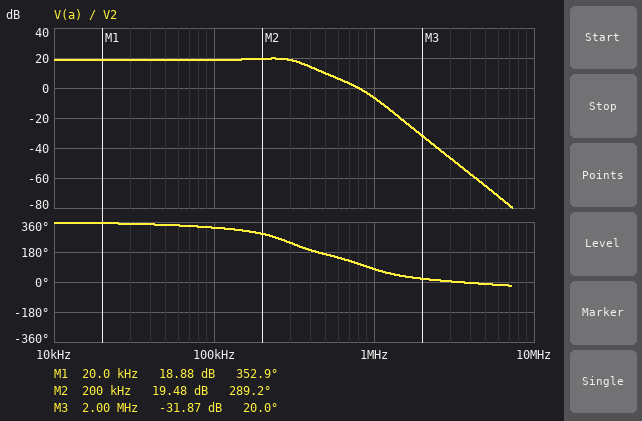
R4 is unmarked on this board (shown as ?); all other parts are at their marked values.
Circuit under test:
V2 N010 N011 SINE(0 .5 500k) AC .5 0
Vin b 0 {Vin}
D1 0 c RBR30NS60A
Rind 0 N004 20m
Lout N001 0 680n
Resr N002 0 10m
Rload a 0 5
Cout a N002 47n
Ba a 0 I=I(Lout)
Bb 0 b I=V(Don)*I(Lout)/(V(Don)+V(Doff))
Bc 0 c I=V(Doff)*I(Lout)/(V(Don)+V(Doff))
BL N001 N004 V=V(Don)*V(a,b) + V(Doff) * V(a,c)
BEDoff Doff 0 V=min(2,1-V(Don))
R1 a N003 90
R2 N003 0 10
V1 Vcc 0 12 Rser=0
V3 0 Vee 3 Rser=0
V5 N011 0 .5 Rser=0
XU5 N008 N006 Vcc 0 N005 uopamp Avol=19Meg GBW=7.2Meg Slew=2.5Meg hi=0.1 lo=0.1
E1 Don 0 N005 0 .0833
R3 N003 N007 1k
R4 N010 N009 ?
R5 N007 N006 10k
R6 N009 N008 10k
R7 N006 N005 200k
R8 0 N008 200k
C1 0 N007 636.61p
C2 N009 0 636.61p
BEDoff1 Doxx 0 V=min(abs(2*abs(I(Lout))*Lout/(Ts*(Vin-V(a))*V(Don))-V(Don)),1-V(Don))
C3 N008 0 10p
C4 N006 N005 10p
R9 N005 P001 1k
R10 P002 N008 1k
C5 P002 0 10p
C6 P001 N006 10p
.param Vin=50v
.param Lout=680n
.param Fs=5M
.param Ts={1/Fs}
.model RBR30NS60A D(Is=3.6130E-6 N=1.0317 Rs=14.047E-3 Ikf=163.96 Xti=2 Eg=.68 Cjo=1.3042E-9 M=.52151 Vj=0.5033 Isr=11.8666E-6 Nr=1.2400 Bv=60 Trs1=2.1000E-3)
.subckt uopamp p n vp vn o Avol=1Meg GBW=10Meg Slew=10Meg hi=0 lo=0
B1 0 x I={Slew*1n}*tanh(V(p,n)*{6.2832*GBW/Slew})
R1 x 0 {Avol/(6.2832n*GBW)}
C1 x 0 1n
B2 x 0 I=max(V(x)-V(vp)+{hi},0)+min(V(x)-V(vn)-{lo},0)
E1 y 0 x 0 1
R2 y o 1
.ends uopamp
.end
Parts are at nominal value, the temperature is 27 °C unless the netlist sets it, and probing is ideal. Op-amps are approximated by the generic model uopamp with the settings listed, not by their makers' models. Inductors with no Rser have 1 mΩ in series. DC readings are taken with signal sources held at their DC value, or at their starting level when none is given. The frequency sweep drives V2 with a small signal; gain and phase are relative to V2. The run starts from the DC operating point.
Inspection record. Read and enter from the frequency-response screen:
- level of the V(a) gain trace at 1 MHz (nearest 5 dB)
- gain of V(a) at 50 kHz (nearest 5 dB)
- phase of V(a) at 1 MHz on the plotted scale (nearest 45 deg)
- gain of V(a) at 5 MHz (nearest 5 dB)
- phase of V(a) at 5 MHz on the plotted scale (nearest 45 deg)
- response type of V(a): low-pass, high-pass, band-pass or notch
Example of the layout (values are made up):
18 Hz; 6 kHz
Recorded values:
-5 dB; 20 dB; 90 deg; -65 dB; 0 deg; low-pass
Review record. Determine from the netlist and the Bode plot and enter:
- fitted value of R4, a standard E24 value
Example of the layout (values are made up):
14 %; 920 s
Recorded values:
1.6 kΩ
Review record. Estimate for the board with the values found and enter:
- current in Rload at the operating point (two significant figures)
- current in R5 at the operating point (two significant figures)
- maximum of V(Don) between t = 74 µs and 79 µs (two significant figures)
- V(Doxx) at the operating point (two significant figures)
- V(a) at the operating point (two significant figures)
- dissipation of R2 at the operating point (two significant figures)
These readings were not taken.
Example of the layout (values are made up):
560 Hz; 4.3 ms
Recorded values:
870 mA; 3.3 µA; 120 mV; 94 mV; 4.4 V; 19 mW
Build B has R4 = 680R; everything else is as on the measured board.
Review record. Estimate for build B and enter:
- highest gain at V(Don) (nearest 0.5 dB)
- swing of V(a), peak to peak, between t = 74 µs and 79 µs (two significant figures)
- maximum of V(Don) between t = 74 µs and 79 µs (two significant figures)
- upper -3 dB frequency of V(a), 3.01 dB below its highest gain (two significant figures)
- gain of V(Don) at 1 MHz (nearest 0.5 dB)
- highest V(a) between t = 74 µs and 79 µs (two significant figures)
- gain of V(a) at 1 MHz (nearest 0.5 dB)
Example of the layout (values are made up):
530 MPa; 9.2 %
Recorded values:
-11.0 dB; 5.9 V; 140 mV; 370 kHz; -34.0 dB; 7.3 V; 0.5 dB
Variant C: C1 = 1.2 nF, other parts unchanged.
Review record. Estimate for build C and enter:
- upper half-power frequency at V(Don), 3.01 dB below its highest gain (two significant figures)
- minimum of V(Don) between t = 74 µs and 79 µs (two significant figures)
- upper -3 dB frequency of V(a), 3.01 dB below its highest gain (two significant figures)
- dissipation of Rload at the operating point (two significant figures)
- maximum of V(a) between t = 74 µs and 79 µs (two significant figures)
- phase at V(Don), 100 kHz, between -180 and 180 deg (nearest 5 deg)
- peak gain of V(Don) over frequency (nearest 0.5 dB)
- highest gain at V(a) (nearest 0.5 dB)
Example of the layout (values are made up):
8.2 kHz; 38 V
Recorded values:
250 kHz; 73 mV; 260 kHz; 3.8 W; 5.6 V; -20 deg; -10.0 dB; 24.0 dB
